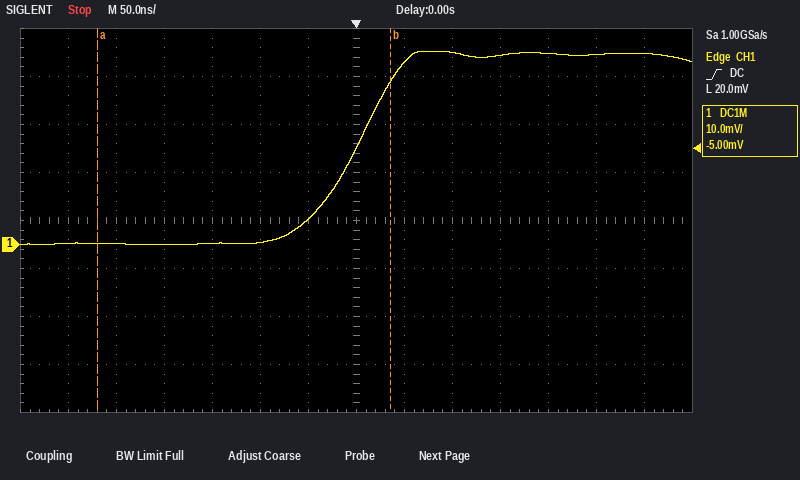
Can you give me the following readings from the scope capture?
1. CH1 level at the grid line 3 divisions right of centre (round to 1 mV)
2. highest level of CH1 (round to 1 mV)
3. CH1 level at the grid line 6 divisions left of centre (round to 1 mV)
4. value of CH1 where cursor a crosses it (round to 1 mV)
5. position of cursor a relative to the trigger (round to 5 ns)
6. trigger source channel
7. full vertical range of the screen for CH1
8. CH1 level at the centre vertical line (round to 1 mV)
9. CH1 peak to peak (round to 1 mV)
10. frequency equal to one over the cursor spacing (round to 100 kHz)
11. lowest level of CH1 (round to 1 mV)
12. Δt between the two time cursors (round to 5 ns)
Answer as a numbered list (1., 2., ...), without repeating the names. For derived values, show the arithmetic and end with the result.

1. 39 mV
2. 40 mV
3. 0 mV
4. 0 mV
5. -270 ns
6. CH1
7. 80 mV
8. 20 mV
9. 40 mV − (0 mV) = 40 mV
10. 1 / 305 ns ≈ 3.3 MHz
11. 0 mV
12. 305 ns
